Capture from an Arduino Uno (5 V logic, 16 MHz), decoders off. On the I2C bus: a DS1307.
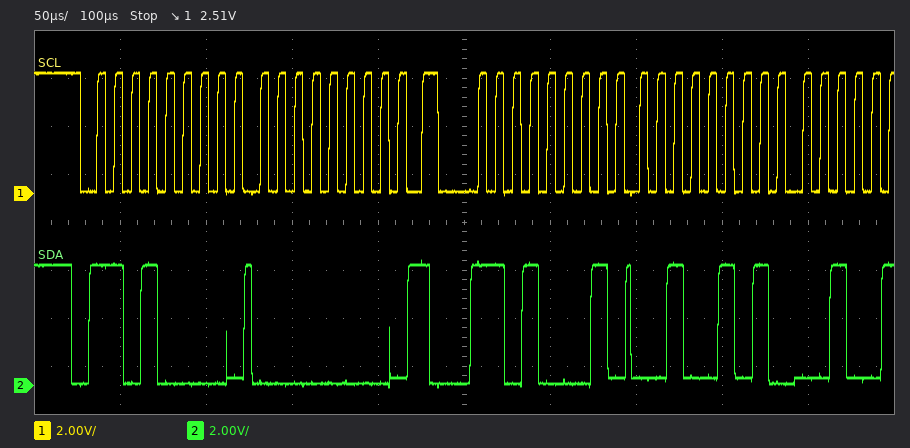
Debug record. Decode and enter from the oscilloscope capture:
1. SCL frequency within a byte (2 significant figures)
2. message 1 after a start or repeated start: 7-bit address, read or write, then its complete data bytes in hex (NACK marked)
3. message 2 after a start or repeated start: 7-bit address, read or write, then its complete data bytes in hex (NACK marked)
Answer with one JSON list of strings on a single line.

["100 kHz", "0x68 write: 00", "0x68 read: 25"]
